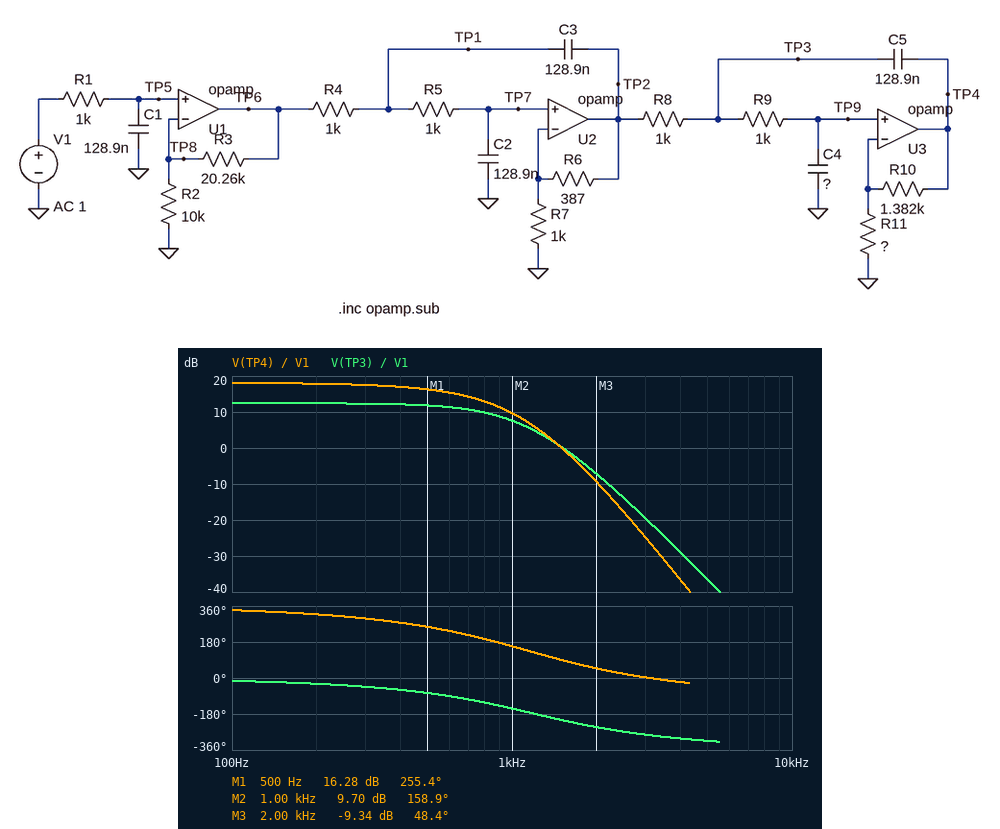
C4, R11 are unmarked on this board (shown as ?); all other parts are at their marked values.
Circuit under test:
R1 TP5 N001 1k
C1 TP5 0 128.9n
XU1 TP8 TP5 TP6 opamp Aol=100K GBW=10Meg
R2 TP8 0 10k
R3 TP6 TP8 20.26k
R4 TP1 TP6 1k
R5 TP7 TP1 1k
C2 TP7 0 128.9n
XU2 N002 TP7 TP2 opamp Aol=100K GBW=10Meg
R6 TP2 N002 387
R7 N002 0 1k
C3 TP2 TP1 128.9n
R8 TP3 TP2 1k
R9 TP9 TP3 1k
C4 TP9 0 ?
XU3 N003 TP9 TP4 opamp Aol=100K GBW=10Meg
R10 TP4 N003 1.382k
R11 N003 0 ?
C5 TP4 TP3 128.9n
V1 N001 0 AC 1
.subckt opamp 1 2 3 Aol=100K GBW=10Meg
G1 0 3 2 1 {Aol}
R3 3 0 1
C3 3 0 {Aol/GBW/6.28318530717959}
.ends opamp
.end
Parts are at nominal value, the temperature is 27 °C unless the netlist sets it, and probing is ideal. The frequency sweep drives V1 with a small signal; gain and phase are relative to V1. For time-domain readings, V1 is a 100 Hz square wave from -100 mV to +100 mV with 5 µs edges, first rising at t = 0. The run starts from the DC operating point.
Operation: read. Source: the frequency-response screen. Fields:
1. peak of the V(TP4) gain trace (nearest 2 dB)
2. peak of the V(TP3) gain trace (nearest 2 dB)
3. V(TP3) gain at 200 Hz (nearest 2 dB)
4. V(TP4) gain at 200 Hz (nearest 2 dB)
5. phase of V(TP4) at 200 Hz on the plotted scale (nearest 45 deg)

18 dB
12 dB
12 dB
18 dB
315 deg
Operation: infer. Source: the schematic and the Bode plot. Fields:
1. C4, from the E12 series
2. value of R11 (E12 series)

180 nF
1.5 kΩ
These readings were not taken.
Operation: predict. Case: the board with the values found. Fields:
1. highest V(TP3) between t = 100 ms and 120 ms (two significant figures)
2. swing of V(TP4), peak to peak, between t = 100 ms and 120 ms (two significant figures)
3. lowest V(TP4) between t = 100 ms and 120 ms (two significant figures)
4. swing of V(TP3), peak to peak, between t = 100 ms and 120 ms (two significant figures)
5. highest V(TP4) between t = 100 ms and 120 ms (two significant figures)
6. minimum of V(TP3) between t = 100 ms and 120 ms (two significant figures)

450 mV
1.6 V
-820 mV
910 mV
820 mV
-450 mV
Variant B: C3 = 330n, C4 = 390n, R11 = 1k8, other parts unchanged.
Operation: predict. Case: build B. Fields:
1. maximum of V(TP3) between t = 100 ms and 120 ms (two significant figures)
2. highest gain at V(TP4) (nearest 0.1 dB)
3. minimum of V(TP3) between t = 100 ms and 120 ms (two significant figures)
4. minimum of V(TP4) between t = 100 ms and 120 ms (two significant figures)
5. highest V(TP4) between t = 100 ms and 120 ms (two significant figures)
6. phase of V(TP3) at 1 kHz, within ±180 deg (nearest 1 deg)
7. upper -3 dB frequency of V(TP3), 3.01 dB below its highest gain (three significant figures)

460 mV
17.4 dB
-460 mV
-740 mV
740 mV
156 deg
854 Hz
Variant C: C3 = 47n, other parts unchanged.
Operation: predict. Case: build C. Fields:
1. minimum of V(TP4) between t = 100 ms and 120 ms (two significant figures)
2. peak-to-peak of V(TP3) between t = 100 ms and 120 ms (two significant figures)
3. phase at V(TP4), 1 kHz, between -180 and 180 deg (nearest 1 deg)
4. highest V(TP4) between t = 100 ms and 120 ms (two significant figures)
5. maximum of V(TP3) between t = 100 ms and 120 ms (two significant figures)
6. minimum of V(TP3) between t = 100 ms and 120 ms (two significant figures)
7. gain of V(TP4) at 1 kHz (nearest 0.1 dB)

-810 mV
840 mV
171 deg
810 mV
420 mV
-420 mV
7.8 dB
